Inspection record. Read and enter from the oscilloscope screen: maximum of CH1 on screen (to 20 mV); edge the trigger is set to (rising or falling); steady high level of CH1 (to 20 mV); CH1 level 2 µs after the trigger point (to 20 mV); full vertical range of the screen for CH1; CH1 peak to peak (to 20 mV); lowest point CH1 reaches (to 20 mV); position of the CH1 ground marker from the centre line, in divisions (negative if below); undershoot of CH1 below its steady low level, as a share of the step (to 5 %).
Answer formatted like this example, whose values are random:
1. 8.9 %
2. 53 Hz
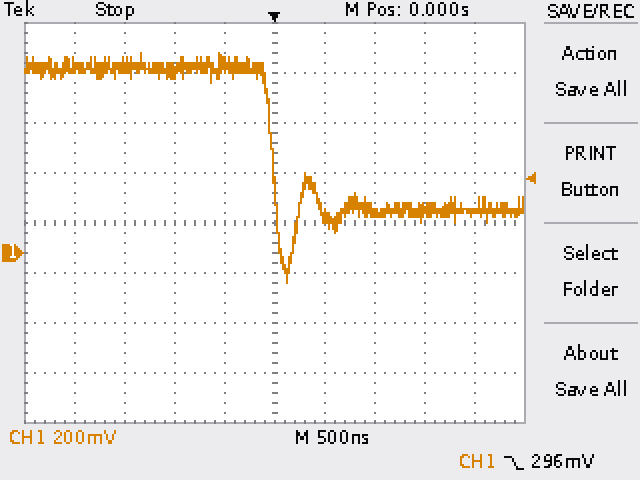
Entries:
1. 800 mV
2. falling
3. 740 mV
4. 160 mV
5. 1.6 V
6. 920 mV
7. -120 mV
8. -0.6 div
9. 50 %
